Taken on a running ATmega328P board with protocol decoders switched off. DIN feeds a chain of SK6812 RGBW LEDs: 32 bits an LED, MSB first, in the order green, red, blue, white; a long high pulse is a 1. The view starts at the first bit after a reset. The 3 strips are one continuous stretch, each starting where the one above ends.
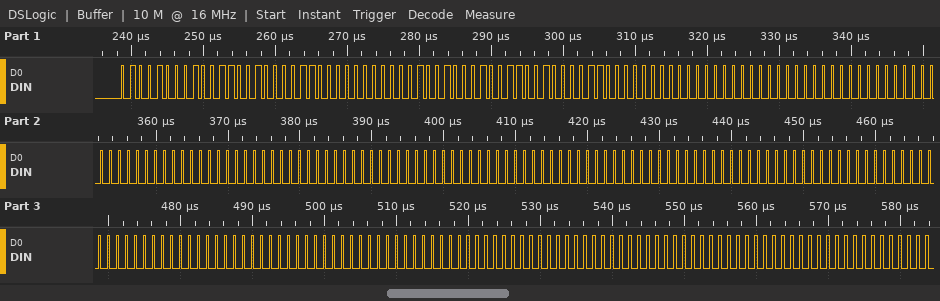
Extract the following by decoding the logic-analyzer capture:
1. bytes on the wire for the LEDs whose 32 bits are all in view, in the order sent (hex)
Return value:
48 99 0C 00 48 99 0C 00 00 00 00 00 00 00 00 00 00 00 00 00 00 00 00 00 00 00 00 00 00 00 00 00
